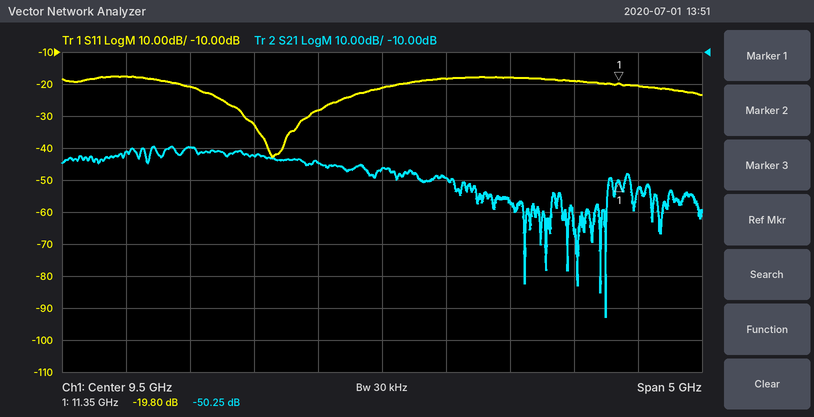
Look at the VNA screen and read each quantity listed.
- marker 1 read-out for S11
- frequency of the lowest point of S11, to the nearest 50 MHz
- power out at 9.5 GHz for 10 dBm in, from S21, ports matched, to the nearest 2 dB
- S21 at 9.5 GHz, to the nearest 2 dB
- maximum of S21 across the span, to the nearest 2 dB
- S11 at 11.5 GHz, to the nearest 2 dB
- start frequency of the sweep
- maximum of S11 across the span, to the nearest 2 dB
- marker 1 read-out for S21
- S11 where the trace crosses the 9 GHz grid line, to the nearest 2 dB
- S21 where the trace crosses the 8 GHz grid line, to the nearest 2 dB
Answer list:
-19.80 dB
8.65 GHz
-36 dBm
-46 dB
-40 dB
-20 dB
7 GHz
-18 dB
-50.25 dB
-28 dB
-40 dB
